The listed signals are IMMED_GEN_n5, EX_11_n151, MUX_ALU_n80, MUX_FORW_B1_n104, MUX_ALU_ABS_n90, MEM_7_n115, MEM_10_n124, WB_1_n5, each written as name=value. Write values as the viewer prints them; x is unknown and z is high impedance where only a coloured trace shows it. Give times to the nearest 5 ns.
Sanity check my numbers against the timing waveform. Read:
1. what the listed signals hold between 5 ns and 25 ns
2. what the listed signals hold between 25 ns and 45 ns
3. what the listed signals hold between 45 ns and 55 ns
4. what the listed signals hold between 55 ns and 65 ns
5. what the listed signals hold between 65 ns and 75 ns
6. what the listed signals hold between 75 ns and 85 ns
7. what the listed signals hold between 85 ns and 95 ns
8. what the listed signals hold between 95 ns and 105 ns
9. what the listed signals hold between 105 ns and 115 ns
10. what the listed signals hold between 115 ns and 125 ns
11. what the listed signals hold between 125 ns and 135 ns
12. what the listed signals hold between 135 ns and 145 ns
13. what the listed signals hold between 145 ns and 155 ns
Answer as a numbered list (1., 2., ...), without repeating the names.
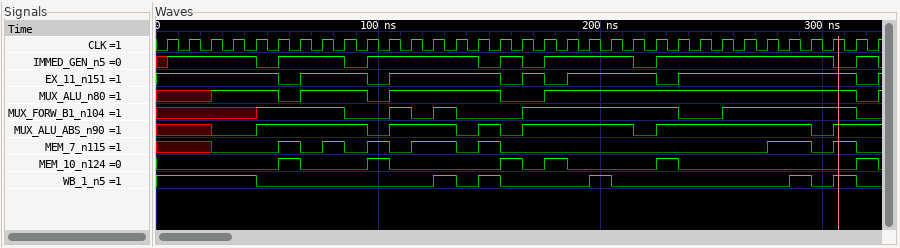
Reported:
1. IMMED_GEN_n5=1, EX_11_n151=1, MUX_ALU_n80=x, MUX_FORW_B1_n104=x, MUX_ALU_ABS_n90=x, MEM_7_n115=x, MEM_10_n124=0, WB_1_n5=1
2. IMMED_GEN_n5=1, EX_11_n151=1, MUX_ALU_n80=1, MUX_FORW_B1_n104=x, MUX_ALU_ABS_n90=0, MEM_7_n115=0, MEM_10_n124=0, WB_1_n5=1
3. IMMED_GEN_n5=0, EX_11_n151=1, MUX_ALU_n80=1, MUX_FORW_B1_n104=1, MUX_ALU_ABS_n90=1, MEM_7_n115=0, MEM_10_n124=0, WB_1_n5=0
4. IMMED_GEN_n5=1, EX_11_n151=0, MUX_ALU_n80=0, MUX_FORW_B1_n104=1, MUX_ALU_ABS_n90=1, MEM_7_n115=1, MEM_10_n124=1, WB_1_n5=0
5. IMMED_GEN_n5=1, EX_11_n151=1, MUX_ALU_n80=1, MUX_FORW_B1_n104=1, MUX_ALU_ABS_n90=1, MEM_7_n115=0, MEM_10_n124=0, WB_1_n5=0
6. IMMED_GEN_n5=1, EX_11_n151=1, MUX_ALU_n80=1, MUX_FORW_B1_n104=1, MUX_ALU_ABS_n90=1, MEM_7_n115=1, MEM_10_n124=0, WB_1_n5=0
7. IMMED_GEN_n5=0, EX_11_n151=1, MUX_ALU_n80=1, MUX_FORW_B1_n104=0, MUX_ALU_ABS_n90=1, MEM_7_n115=0, MEM_10_n124=0, WB_1_n5=0
8. IMMED_GEN_n5=1, EX_11_n151=0, MUX_ALU_n80=0, MUX_FORW_B1_n104=0, MUX_ALU_ABS_n90=0, MEM_7_n115=1, MEM_10_n124=1, WB_1_n5=0
9. IMMED_GEN_n5=1, EX_11_n151=1, MUX_ALU_n80=1, MUX_FORW_B1_n104=1, MUX_ALU_ABS_n90=1, MEM_7_n115=0, MEM_10_n124=0, WB_1_n5=0
10. IMMED_GEN_n5=1, EX_11_n151=1, MUX_ALU_n80=1, MUX_FORW_B1_n104=0, MUX_ALU_ABS_n90=1, MEM_7_n115=1, MEM_10_n124=0, WB_1_n5=0
11. IMMED_GEN_n5=1, EX_11_n151=1, MUX_ALU_n80=1, MUX_FORW_B1_n104=1, MUX_ALU_ABS_n90=1, MEM_7_n115=1, MEM_10_n124=0, WB_1_n5=1
12. IMMED_GEN_n5=1, EX_11_n151=1, MUX_ALU_n80=1, MUX_FORW_B1_n104=0, MUX_ALU_ABS_n90=0, MEM_7_n115=0, MEM_10_n124=0, WB_1_n5=0
13. IMMED_GEN_n5=0, EX_11_n151=1, MUX_ALU_n80=1, MUX_FORW_B1_n104=0, MUX_ALU_ABS_n90=1, MEM_7_n115=1, MEM_10_n124=0, WB_1_n5=1
